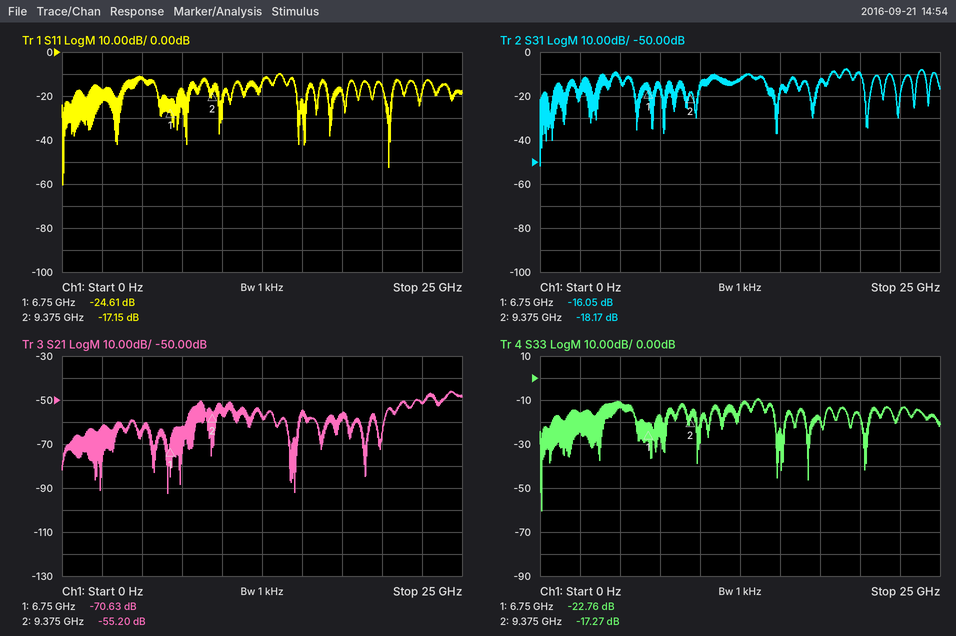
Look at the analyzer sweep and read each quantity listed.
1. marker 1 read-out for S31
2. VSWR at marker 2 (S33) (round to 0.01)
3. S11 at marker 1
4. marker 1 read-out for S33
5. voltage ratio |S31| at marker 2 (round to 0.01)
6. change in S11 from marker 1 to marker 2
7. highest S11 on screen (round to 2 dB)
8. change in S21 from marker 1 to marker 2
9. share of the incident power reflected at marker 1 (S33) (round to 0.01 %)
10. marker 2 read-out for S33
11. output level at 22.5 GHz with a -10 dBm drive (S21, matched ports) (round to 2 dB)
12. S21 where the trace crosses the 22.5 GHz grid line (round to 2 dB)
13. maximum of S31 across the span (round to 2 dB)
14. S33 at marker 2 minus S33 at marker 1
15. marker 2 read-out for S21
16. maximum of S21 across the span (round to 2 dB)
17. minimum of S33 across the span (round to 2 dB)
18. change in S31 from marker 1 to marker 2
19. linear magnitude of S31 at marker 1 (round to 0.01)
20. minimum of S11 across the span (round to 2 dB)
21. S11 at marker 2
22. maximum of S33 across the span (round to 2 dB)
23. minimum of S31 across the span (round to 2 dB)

-16.05 dB
1.32
-24.61 dB
-22.76 dB
0.12
7.46 dB
-10 dB
15.43 dB
0.53 %
-17.27 dB
-62 dBm
-52 dB
-8 dB
5.49 dB
-55.20 dB
-46 dB
-60 dB
-2.12 dB
0.16
-60 dB
-17.15 dB
-10 dB
-52 dB
